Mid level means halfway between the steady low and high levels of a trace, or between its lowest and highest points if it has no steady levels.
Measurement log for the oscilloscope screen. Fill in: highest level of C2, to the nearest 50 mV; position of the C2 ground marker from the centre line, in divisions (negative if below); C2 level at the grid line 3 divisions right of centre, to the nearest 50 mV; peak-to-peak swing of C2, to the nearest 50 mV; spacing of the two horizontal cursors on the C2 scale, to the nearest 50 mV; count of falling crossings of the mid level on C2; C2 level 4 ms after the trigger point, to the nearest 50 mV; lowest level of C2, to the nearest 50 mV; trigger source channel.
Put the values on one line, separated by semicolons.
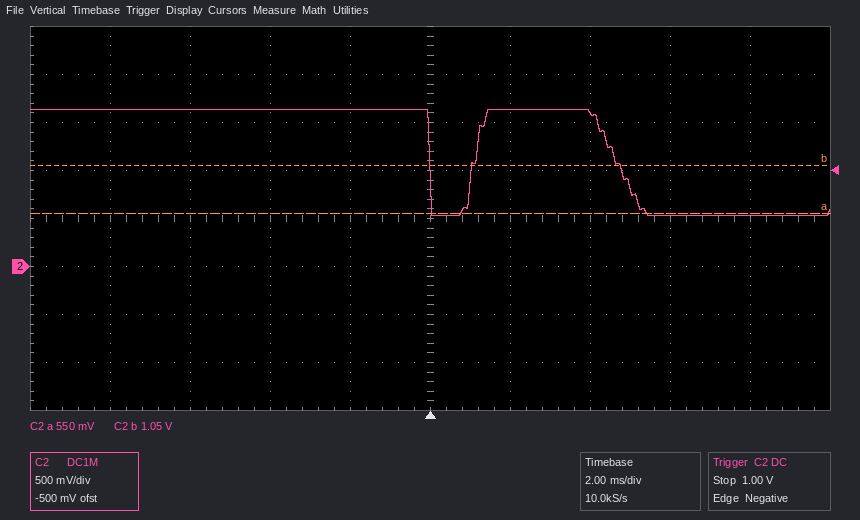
1.65 V; -1.0 div; 550 mV; 1.10 V; 500 mV; 2; 1.60 V; 550 mV; C2
